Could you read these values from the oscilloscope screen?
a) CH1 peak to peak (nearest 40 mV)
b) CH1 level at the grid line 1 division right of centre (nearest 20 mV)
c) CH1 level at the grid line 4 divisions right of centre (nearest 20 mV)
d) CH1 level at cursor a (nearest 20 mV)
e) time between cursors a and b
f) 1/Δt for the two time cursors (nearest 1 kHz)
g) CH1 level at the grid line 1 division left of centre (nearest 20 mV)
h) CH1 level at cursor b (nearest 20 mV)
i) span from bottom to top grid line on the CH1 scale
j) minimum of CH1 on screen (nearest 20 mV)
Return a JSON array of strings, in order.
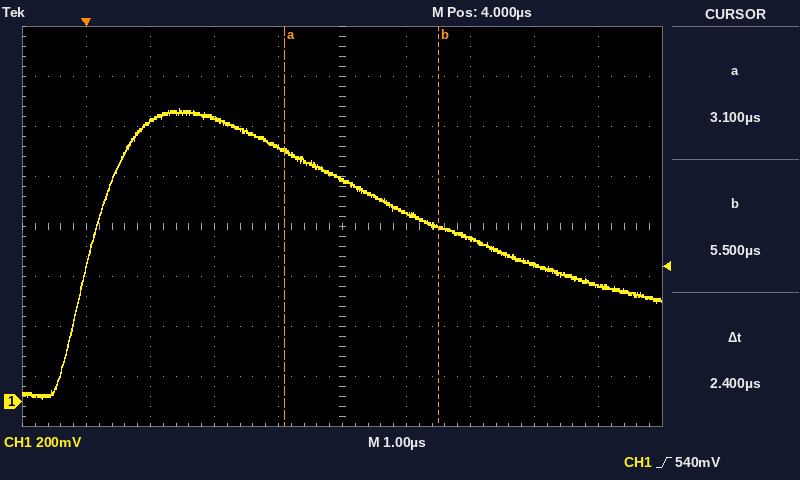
["1.16 V", "760 mV", "460 mV", "1.00 V", "2.4 µs", "417 kHz", "1.02 V", "700 mV", "1.6 V", "20 mV"]
